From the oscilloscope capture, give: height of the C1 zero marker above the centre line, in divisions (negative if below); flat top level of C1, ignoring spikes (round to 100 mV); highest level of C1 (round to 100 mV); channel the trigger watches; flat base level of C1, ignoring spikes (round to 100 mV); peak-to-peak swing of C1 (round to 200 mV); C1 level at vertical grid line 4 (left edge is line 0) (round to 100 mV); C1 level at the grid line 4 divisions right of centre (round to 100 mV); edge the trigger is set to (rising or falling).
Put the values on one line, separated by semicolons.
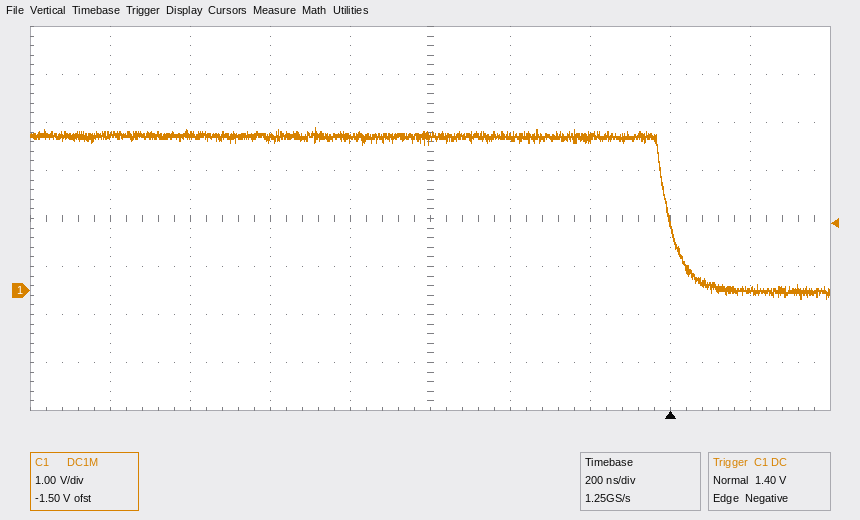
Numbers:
-1.5 div; 3.2 V; 3.4 V; C1; 0.0 V; 3.6 V; 3.2 V; 0.0 V; falling
